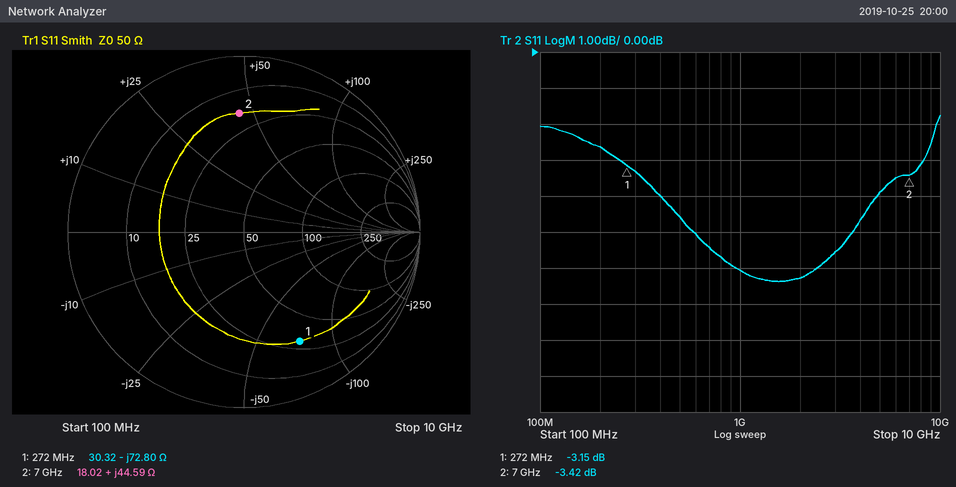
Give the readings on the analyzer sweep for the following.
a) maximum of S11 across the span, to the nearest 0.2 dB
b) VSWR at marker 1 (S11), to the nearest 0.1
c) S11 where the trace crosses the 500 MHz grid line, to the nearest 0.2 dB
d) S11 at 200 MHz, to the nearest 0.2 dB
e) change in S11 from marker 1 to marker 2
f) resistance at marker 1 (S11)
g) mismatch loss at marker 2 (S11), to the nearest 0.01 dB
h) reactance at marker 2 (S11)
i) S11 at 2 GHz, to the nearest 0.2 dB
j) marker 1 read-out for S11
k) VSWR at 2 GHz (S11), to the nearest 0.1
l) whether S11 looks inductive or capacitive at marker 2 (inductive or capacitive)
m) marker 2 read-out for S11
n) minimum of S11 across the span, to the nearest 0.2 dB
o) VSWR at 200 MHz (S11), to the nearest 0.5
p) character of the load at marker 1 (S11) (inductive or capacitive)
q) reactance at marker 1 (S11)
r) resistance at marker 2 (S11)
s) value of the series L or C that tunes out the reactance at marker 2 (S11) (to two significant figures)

-1.8 dB
5.6
-4.6 dB
-2.6 dB
-0.27 dB
30.32 Ω
2.64 dB
+44.59 Ω
-6.2 dB
-3.15 dB
2.9
inductive
-3.42 dB
-6.4 dB
6.5
capacitive
-72.80 Ω
18.02 Ω
510 fF
